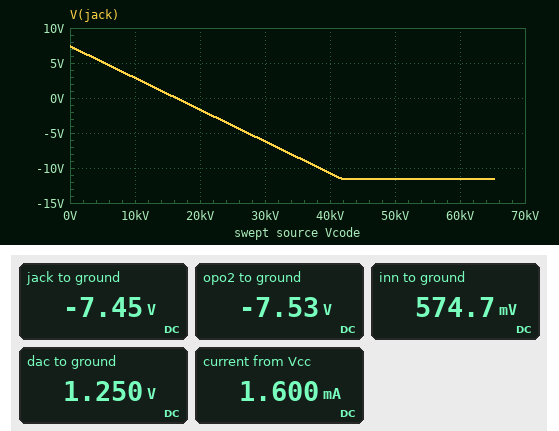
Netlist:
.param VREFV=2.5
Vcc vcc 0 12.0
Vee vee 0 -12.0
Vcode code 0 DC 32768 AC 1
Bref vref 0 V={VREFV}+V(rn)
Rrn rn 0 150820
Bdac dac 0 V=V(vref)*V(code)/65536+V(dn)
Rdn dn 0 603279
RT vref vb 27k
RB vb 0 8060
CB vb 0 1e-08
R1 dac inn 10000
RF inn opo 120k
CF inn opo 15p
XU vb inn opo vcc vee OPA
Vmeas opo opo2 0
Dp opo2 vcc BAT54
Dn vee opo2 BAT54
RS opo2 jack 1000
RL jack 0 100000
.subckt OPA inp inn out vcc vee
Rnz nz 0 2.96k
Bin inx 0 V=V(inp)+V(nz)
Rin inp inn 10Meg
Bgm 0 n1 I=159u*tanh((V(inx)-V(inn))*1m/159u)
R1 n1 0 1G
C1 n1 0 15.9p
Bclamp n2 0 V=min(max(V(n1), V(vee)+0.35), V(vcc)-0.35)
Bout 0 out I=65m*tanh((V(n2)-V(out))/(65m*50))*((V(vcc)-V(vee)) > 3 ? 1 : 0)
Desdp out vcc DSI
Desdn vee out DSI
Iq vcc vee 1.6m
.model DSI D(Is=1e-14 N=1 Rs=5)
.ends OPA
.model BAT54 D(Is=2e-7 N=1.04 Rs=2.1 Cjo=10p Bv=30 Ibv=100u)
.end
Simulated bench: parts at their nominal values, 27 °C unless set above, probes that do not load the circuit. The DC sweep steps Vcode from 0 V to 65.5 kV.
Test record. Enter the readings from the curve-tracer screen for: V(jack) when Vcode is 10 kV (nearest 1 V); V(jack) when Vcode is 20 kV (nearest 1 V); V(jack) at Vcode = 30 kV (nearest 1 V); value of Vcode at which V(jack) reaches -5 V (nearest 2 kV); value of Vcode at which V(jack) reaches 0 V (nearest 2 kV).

3 V
-2 V
-6 V
28 kV
16 kV
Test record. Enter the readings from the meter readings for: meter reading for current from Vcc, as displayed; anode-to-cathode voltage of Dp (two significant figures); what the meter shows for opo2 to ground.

1.600 mA
-20 V
-7.53 V
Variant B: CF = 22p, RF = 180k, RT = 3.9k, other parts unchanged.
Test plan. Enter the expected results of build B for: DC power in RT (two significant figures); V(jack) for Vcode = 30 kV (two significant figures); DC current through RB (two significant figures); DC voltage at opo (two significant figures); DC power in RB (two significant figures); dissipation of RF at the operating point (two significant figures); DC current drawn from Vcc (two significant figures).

170 µW
11 V
210 µA
9.5 V
350 µW
340 µW
1.6 mA
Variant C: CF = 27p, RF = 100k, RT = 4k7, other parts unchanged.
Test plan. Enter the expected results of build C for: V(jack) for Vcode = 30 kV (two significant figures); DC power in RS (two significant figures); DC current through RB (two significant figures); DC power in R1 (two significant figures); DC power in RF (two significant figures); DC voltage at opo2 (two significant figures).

5.9 V
2.3 µW
200 µA
11 µW
110 µW
4.9 V
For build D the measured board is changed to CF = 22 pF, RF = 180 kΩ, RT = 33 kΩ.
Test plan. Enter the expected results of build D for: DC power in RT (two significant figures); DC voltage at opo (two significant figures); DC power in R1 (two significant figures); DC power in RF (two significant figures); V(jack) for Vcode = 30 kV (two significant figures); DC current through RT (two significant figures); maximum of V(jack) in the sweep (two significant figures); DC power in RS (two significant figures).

120 µW
-12 V
46 µW
830 µW
-11 V
61 µA
9.2 V
13 µW
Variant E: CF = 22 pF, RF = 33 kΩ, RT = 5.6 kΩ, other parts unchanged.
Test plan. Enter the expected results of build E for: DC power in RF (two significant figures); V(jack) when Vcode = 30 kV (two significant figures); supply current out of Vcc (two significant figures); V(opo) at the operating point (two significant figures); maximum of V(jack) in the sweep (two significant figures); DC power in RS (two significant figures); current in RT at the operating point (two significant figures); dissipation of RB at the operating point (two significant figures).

17 µW
2.5 V
1.6 mA
2.2 V
6.3 V
480 nW
180 µA
270 µW
